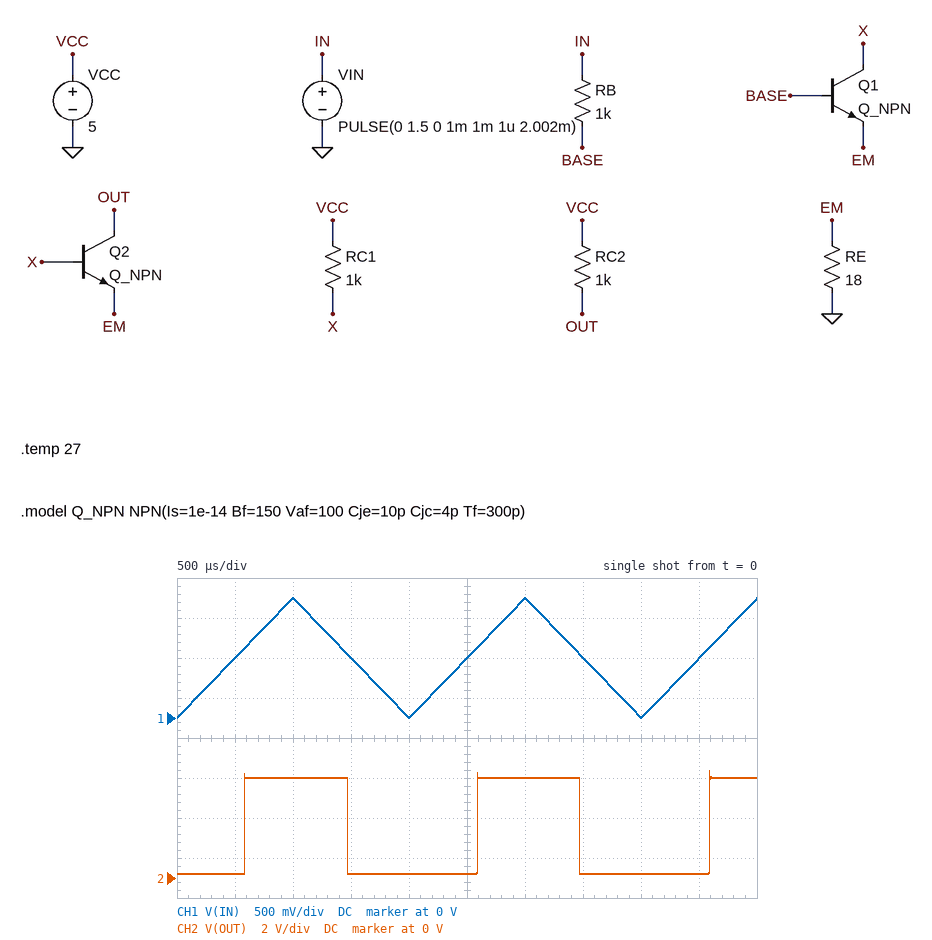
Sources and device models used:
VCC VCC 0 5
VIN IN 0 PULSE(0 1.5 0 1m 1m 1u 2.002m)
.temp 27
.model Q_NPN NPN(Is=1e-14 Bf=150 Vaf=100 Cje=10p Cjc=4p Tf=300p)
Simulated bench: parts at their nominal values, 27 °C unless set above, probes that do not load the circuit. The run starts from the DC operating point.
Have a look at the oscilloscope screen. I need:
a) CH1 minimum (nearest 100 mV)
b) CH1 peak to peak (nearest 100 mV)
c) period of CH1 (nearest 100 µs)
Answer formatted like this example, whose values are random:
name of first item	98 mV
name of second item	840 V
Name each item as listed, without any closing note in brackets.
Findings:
CH1 minimum	0 V
CH1 peak to peak	1.5 V
period of CH1	2.0 ms
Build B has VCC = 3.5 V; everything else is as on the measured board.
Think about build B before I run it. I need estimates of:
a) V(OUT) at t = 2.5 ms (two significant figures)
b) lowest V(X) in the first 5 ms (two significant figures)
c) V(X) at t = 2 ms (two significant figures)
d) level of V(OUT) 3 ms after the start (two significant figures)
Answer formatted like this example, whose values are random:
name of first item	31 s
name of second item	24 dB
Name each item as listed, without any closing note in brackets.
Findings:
V(OUT) at t = 2.5 ms	140 mV
lowest V(X) in the first 5 ms	120 mV
V(X) at t = 2 ms	820 mV
level of V(OUT) 3 ms after the start	3.5 V
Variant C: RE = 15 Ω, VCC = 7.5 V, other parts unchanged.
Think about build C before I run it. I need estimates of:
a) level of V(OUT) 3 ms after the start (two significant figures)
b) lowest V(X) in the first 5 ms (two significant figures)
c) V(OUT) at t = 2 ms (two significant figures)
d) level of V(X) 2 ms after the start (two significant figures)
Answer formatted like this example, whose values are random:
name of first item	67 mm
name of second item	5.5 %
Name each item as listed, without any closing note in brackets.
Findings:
level of V(OUT) 3 ms after the start	7.5 V
lowest V(X) in the first 5 ms	190 mV
V(OUT) at t = 2 ms	240 mV
level of V(X) 2 ms after the start	940 mV
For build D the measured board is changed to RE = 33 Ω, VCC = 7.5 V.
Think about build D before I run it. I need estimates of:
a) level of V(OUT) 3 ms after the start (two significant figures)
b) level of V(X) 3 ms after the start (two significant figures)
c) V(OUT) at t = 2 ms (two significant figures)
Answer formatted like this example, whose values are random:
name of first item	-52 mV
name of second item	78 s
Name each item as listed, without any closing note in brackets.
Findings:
level of V(OUT) 3 ms after the start	7.5 V
level of V(X) 3 ms after the start	330 mV
V(OUT) at t = 2 ms	470 mV
